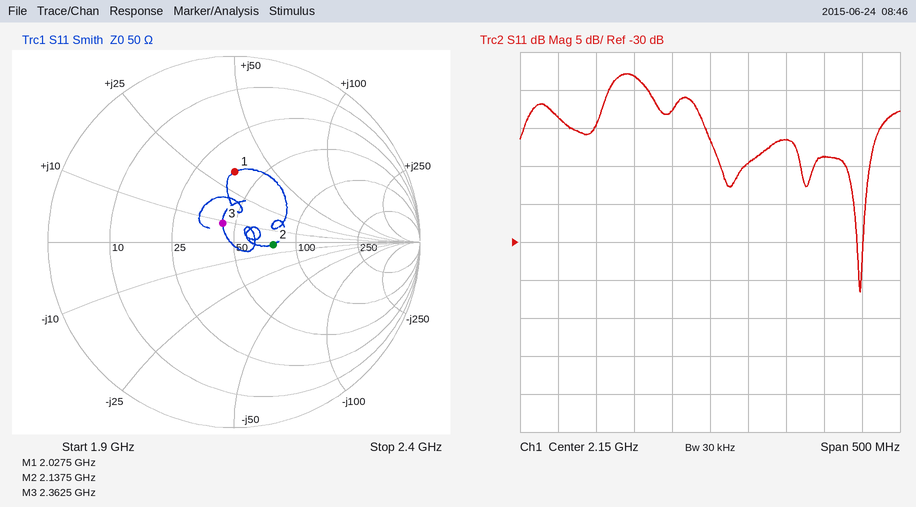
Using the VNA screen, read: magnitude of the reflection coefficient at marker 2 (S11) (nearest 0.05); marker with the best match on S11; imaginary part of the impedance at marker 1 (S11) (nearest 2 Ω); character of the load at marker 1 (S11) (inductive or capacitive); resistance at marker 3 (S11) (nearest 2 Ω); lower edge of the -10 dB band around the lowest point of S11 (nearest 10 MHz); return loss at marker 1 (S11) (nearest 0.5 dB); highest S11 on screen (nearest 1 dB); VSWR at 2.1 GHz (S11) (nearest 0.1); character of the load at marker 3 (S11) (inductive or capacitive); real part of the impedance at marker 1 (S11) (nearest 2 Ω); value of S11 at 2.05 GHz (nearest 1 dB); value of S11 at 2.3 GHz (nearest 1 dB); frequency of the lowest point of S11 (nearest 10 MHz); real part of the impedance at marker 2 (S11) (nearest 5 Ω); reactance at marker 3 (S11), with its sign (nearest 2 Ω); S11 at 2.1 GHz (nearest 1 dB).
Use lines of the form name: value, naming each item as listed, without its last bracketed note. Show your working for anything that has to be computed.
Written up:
magnitude of the reflection coefficient at marker 2 (S11): 0.20
marker with the best match on S11: marker 3
imaginary part of the impedance at marker 1 (S11): +34 Ω
character of the load at marker 1 (S11): inductive
resistance at marker 3 (S11): 44 Ω
lower edge of the -10 dB band around the lowest point of S11: 2.07 GHz
return loss at marker 1 (S11): 8.5 dB
highest S11 on screen: -8 dB
VSWR at 2.1 GHz (S11): |Γ| = 10^(-13/20) = 0.2239; VSWR = (1 + 0.2239)/(1 − 0.2239) ≈ 1.6
character of the load at marker 3 (S11): inductive
real part of the impedance at marker 1 (S11): 38 Ω
value of S11 at 2.05 GHz: -8 dB
value of S11 at 2.3 GHz: -19 dB
frequency of the lowest point of S11: 2.35 GHz
real part of the impedance at marker 2 (S11): 75 Ω
reactance at marker 3 (S11), with its sign: +8 Ω
S11 at 2.1 GHz: -13 dB
